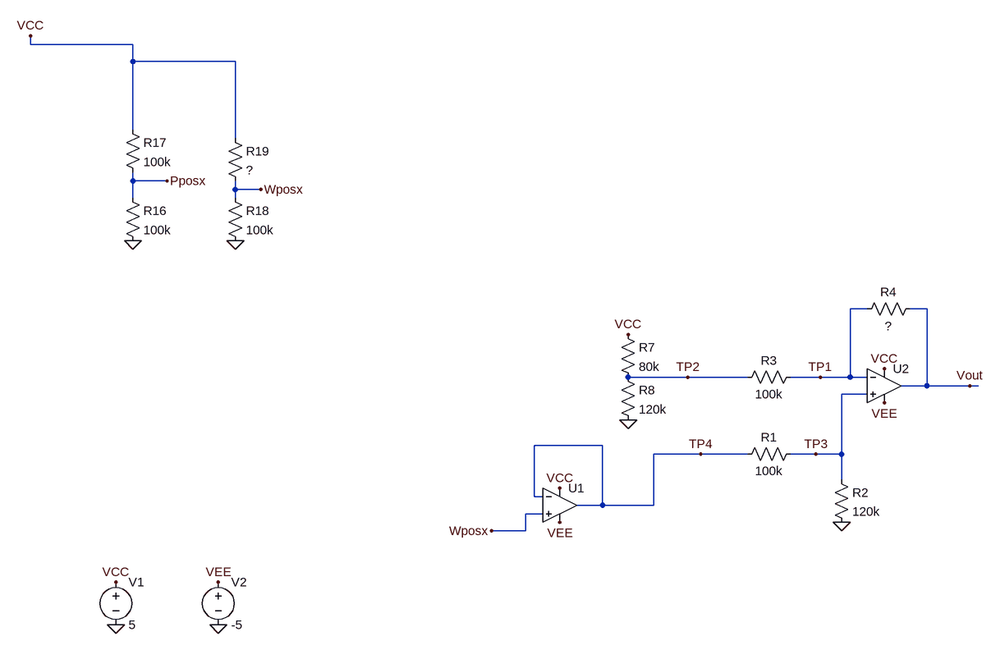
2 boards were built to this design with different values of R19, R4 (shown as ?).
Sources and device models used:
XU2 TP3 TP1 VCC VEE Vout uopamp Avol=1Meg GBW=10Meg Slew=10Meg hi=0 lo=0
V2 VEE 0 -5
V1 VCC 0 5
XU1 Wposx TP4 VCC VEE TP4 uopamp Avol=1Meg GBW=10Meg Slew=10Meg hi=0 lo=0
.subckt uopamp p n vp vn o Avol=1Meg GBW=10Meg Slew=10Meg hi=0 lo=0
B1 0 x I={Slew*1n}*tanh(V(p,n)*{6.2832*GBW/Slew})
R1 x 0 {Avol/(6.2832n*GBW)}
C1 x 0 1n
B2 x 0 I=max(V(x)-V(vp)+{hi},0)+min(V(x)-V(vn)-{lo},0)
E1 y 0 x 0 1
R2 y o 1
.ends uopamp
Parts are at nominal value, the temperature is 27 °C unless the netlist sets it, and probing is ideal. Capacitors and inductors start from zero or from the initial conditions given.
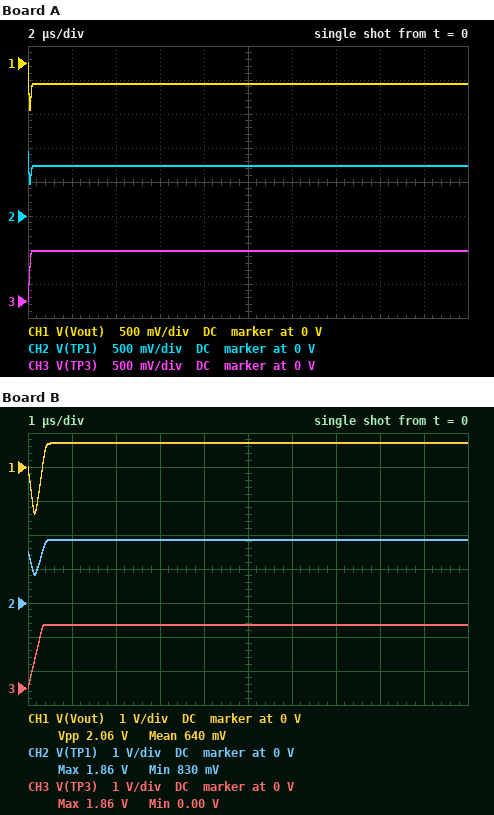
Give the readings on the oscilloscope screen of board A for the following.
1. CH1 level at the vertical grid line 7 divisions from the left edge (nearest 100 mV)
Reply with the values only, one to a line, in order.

-300 mV
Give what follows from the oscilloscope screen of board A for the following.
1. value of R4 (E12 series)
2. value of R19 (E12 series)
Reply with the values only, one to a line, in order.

68 kΩ
270 kΩ
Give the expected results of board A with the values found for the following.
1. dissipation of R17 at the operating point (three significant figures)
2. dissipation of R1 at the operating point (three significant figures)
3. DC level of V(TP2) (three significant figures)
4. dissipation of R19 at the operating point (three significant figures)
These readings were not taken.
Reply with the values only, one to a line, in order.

62.5 µW
3.77 µW
2.27 V
49.3 µW
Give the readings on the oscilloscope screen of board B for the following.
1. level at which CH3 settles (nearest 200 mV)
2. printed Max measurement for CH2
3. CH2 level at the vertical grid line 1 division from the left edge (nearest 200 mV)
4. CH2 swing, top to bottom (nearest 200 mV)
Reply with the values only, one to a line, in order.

1.8 V
1.86 V
1.8 V
1.0 V
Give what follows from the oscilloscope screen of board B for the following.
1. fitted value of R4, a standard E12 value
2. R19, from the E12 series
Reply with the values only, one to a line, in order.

150 kΩ
47 kΩ
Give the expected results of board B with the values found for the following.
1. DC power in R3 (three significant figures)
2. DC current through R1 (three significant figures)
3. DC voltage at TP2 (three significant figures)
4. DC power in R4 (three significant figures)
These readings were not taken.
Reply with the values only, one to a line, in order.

5.98 µW
15.5 µA
2.63 V
8.97 µW
